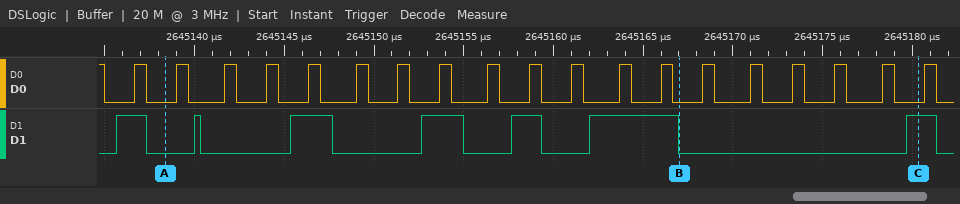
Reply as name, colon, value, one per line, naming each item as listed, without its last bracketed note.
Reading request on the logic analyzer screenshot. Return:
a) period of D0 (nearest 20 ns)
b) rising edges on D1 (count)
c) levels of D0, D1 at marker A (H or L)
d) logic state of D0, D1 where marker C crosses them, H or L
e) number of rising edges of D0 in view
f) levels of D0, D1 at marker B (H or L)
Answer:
period of D0: 2440 ns
rising edges on D1: 7
levels of D0, D1 at marker A: D0=L, D1=L
logic state of D0, D1 where marker C crosses them, H or L: D0=L, D1=H
number of rising edges of D0 in view: 19
levels of D0, D1 at marker B: D0=L, D1=L
